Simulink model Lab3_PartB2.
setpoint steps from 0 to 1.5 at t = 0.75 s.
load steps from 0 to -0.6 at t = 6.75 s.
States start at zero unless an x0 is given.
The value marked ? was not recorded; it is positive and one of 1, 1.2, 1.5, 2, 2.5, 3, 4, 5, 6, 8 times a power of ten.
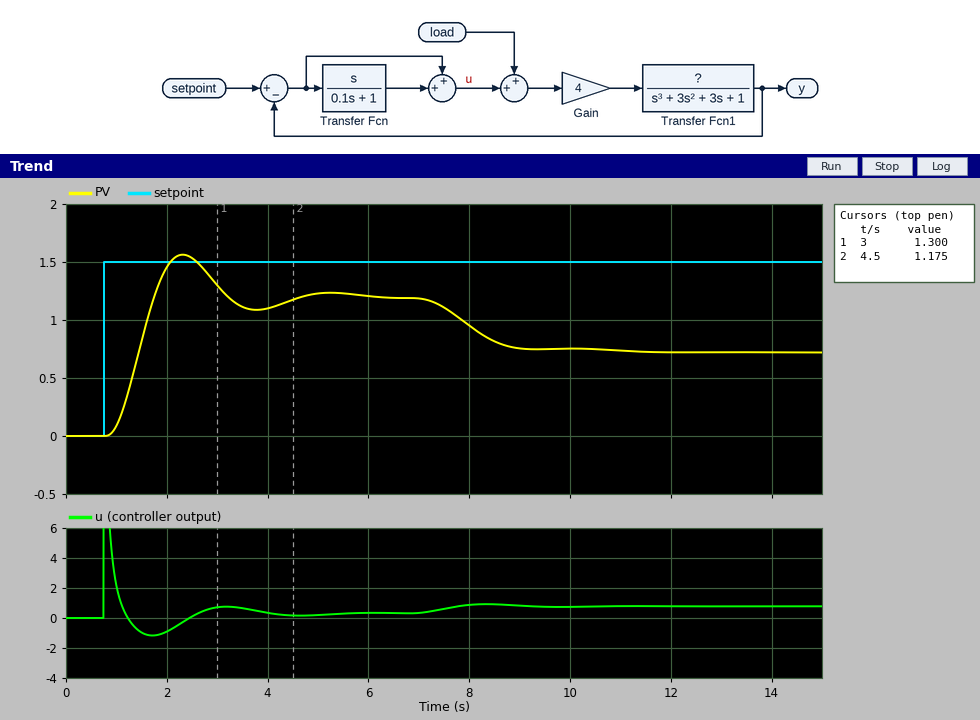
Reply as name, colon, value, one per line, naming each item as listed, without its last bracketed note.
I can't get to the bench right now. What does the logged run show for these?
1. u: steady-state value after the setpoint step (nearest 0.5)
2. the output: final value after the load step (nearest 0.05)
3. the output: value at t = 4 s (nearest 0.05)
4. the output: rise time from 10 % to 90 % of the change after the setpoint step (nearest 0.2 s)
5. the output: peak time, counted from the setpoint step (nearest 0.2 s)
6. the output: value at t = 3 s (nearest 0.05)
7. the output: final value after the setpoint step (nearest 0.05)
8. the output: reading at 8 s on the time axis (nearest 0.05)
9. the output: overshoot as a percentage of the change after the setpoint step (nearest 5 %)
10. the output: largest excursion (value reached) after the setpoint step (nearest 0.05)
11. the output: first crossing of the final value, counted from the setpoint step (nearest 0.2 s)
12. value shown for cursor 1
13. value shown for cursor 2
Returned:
u: steady-state value after the setpoint step: 0.5
the output: final value after the load step: 0.70
the output: value at t = 4 s: 1.10
the output: rise time from 10 % to 90 % of the change after the setpoint step: 0.6 s
the output: peak time, counted from the setpoint step: 1.6 s
the output: value at t = 3 s: 1.30
the output: final value after the setpoint step: 1.20
the output: reading at 8 s on the time axis: 0.95
the output: overshoot as a percentage of the change after the setpoint step: 30 %
the output: largest excursion (value reached) after the setpoint step: 1.55
the output: first crossing of the final value, counted from the setpoint step: 1.0 s
value shown for cursor 1: 1.300
value shown for cursor 2: 1.175
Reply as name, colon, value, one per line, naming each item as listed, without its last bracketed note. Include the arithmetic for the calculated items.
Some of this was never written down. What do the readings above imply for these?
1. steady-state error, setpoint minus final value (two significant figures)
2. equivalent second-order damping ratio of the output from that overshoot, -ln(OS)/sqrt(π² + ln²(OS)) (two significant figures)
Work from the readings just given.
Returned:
steady-state error, setpoint minus final value: 1.5 - 1.2 = 0.30
equivalent second-order damping ratio of the output from that overshoot, -ln(OS)/sqrt(π² + ln²(OS)): ln(0.3) = -1.204; 1.204 / sqrt(9.870 + 1.450) = 0.36
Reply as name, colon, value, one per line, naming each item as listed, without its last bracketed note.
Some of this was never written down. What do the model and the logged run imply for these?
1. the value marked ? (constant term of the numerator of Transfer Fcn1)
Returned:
the value marked ?: 1
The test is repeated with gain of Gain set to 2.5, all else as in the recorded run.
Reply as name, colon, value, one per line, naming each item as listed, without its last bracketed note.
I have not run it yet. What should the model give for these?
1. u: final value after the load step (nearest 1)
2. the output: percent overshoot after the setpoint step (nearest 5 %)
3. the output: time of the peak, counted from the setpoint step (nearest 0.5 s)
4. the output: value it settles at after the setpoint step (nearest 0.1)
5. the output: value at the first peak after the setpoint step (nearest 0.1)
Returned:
u: final value after the load step: 1
the output: percent overshoot after the setpoint step: 20 %
the output: time of the peak, counted from the setpoint step: 2.0 s
the output: value it settles at after the setpoint step: 1.1
the output: value at the first peak after the setpoint step: 1.3
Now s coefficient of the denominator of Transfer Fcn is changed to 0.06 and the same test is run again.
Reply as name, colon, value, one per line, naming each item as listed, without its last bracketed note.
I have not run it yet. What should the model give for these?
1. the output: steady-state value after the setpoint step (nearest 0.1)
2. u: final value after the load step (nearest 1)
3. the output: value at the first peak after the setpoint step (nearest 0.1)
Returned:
the output: steady-state value after the setpoint step: 1.2
u: final value after the load step: 1
the output: value at the first peak after the setpoint step: 1.5
